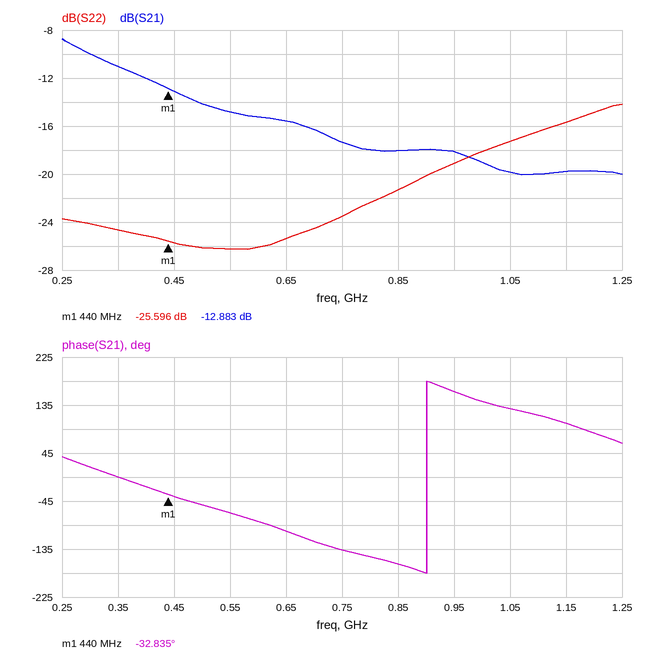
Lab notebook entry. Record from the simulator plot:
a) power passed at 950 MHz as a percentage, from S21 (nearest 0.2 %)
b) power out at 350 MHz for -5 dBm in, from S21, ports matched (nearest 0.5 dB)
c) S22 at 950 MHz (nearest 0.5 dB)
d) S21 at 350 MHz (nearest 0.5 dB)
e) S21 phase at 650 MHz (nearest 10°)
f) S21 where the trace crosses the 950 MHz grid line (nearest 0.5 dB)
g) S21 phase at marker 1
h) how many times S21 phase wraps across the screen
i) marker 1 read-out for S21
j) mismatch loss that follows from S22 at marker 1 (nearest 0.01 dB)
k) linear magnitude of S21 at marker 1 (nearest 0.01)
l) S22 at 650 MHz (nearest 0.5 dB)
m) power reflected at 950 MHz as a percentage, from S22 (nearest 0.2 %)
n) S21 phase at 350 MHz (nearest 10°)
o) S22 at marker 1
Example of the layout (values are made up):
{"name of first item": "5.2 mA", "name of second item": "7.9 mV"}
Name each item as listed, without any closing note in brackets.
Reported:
{"power passed at 950 MHz as a percentage, from S21": "1.6 %", "power out at 350 MHz for -5 dBm in, from S21, ports matched": "-16.0 dBm", "S22 at 950 MHz": "-19.0 dB", "S21 at 350 MHz": "-11.0 dB", "S21 phase at 650 MHz": "-100°", "S21 where the trace crosses the 950 MHz grid line": "-18.0 dB", "S21 phase at marker 1": "-32.835°", "how many times S21 phase wraps across the screen": "1", "marker 1 read-out for S21": "-12.883 dB", "mismatch loss that follows from S22 at marker 1": "0.01 dB", "linear magnitude of S21 at marker 1": "0.23", "S22 at 650 MHz": "-25.5 dB", "power reflected at 950 MHz as a percentage, from S22": "1.2 %", "S21 phase at 350 MHz": "0°", "S22 at marker 1": "-25.596 dB"}
